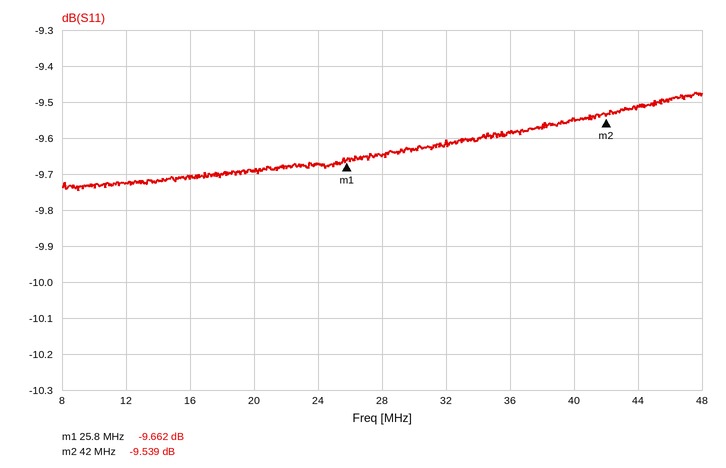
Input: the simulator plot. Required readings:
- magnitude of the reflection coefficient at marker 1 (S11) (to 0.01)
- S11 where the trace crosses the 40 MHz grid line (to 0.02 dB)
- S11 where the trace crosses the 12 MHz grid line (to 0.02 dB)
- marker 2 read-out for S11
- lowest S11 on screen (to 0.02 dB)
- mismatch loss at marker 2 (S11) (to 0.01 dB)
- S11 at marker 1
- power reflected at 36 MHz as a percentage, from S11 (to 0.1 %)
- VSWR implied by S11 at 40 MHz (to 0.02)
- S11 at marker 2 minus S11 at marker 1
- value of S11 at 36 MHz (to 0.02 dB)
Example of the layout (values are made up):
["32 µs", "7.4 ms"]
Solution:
["0.33", "-9.54 dB", "-9.72 dB", "-9.539 dB", "-9.74 dB", "0.51 dB", "-9.662 dB", "11.0 %", "2.00", "0.123 dB", "-9.58 dB"]
